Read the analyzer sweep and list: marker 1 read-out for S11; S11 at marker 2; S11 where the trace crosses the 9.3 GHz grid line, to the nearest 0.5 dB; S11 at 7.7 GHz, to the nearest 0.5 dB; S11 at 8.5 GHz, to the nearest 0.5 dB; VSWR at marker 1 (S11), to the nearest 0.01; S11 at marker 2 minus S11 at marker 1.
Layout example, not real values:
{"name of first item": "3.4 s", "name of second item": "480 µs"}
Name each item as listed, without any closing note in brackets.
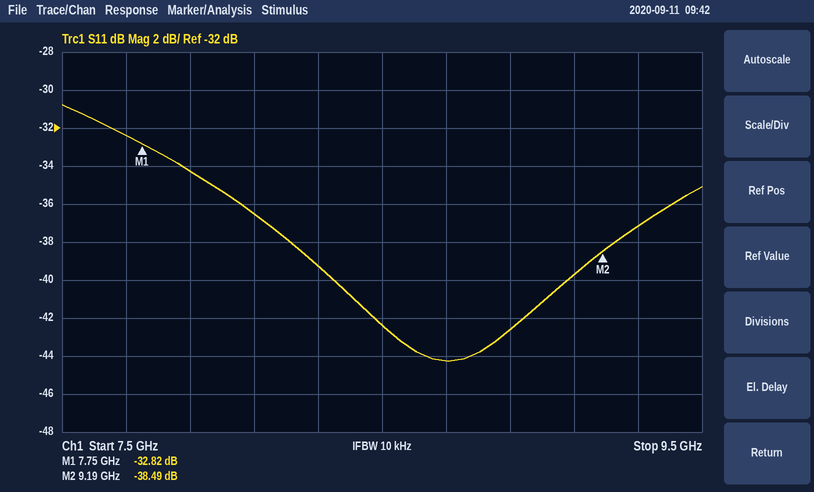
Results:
{"marker 1 read-out for S11": "-32.82 dB", "S11 at marker 2": "-38.49 dB", "S11 where the trace crosses the 9.3 GHz grid line, to the nearest 0.5 dB": "-37.0 dB", "S11 at 7.7 GHz, to the nearest 0.5 dB": "-32.5 dB", "S11 at 8.5 GHz, to the nearest 0.5 dB": "-42.5 dB", "VSWR at marker 1 (S11), to the nearest 0.01": "1.05", "S11 at marker 2 minus S11 at marker 1": "-5.67 dB"}
